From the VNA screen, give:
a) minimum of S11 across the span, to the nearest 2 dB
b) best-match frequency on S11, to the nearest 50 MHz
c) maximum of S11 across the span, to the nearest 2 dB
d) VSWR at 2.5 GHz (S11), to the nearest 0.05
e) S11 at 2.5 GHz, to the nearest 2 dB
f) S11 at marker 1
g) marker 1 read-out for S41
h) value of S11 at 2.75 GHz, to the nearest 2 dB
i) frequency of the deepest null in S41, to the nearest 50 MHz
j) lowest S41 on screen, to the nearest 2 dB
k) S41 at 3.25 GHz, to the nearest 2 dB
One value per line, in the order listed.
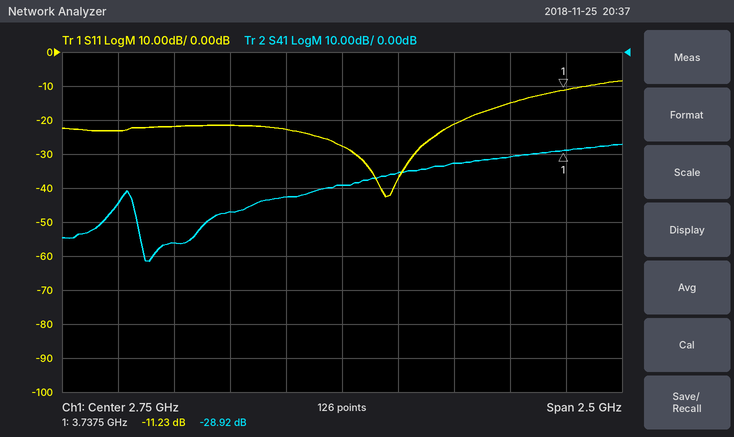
-42 dB
2.95 GHz
-8 dB
1.15
-22 dB
-11.23 dB
-28.92 dB
-28 dB
1.90 GHz
-62 dB
-32 dB
